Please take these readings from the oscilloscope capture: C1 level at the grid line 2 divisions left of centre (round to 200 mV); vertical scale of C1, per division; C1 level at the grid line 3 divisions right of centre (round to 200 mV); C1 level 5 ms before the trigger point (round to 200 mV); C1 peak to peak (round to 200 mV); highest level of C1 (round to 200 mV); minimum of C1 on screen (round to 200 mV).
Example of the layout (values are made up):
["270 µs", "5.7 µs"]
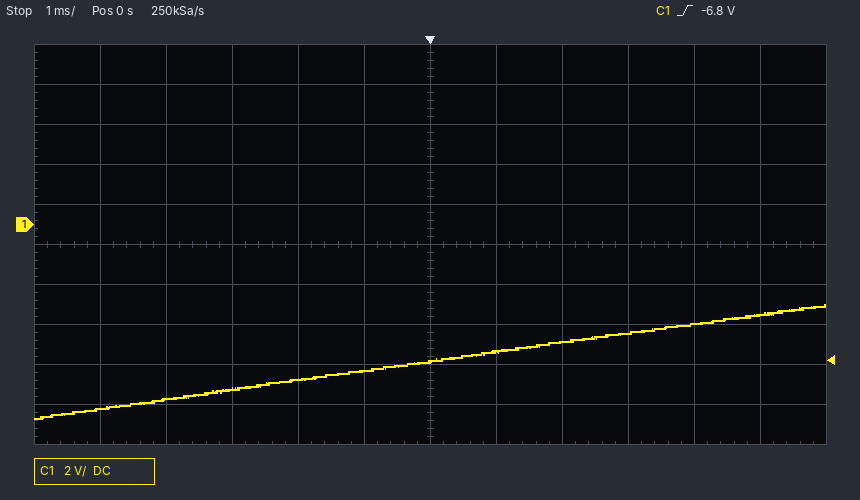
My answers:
["-7.8 V", "2 V", "-5.4 V", "-9.2 V", "5.6 V", "-4.0 V", "-9.6 V"]
